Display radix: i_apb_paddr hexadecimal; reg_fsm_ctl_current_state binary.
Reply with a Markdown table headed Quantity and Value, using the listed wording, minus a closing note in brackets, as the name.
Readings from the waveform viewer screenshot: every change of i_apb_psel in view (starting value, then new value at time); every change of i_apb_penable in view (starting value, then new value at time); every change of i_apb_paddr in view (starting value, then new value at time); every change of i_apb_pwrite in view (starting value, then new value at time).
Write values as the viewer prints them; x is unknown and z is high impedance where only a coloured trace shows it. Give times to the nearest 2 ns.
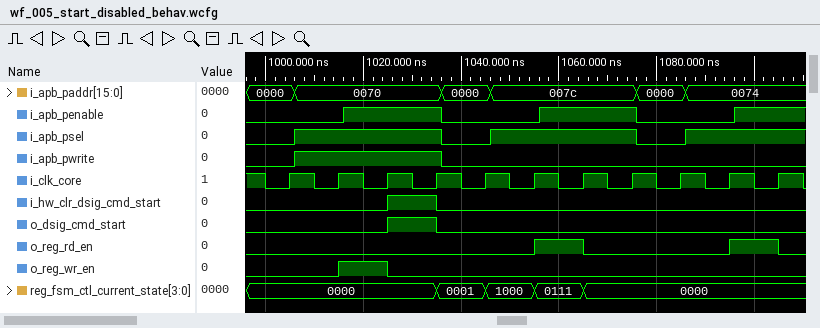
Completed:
| Quantity | Value |
|---|---|
| every change of i_apb_psel in view | 0, 1 at 1006 ns, 0 at 1036 ns, 1 at 1046 ns, 0 at 1076 ns, 1 at 1086 ns |
| every change of i_apb_penable in view | 0, 1 at 1016 ns, 0 at 1036 ns, 1 at 1056 ns, 0 at 1076 ns, 1 at 1096 ns |
| every change of i_apb_paddr in view | 0000, 0070 at 1006 ns, 0000 at 1036 ns, 007c at 1046 ns, 0000 at 1076 ns, 0074 at 1086 ns |
| every change of i_apb_pwrite in view | 0, 1 at 1006 ns, 0 at 1036 ns |
